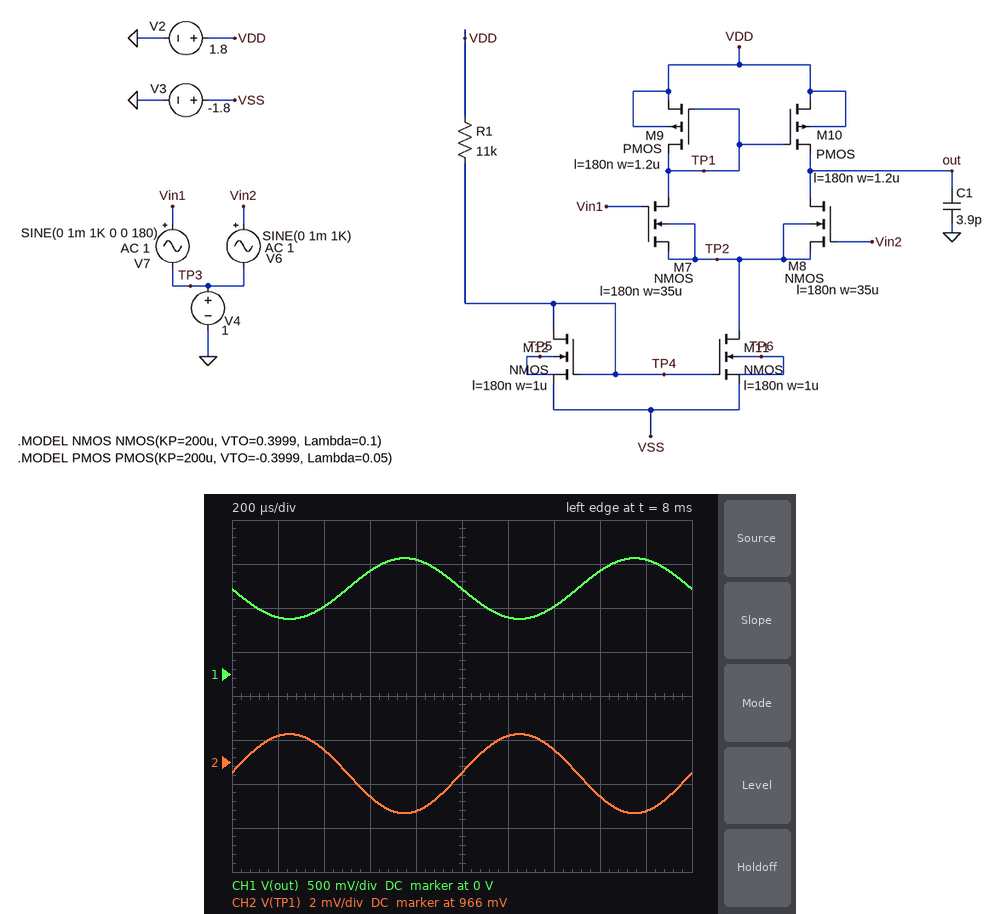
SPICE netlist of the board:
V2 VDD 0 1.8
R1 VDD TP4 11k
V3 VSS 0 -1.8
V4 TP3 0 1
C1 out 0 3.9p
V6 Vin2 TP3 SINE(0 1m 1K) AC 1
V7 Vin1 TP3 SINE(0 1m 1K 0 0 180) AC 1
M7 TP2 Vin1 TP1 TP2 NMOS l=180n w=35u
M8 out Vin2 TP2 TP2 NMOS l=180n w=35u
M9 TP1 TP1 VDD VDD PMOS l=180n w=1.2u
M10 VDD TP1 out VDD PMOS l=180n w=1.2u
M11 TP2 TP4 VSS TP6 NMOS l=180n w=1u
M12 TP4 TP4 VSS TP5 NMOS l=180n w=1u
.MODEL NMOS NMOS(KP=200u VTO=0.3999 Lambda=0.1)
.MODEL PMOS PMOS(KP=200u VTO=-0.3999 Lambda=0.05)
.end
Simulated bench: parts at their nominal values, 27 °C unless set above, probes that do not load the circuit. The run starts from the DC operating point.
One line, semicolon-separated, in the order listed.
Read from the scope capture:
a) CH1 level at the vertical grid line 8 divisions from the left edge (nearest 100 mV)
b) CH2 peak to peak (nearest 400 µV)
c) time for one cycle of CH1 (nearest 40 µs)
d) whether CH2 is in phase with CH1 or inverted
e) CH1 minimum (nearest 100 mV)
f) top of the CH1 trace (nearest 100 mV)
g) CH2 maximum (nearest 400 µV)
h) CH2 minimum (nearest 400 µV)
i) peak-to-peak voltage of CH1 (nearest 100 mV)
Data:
1.2 V; 3.6 mV; 1.00 ms; inverted; 600 mV; 1.3 V; 967.2 mV; 963.6 mV; 700 mV
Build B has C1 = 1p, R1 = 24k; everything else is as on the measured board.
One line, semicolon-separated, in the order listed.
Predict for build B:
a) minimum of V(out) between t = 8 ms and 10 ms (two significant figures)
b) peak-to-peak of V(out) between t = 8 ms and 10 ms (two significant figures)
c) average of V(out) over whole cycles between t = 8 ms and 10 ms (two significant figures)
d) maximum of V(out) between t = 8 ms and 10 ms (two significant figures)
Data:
610 mV; 910 mV; 1.1 V; 1.5 V
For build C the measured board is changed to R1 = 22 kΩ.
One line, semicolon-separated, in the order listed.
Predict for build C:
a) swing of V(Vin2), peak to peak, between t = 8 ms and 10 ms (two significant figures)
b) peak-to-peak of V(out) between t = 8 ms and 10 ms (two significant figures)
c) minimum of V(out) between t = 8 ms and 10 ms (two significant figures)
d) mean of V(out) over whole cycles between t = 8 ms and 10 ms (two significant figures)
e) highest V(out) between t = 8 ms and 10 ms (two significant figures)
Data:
2.0 mV; 890 mV; 620 mV; 1.1 V; 1.5 V
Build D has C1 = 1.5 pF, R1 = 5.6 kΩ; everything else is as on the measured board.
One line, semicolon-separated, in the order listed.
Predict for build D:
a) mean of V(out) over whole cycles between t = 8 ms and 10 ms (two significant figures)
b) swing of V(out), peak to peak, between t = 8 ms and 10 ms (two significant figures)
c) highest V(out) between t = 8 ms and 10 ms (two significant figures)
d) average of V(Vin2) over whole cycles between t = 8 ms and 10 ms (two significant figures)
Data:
830 mV; 490 mV; 1.1 V; 1.0 V
